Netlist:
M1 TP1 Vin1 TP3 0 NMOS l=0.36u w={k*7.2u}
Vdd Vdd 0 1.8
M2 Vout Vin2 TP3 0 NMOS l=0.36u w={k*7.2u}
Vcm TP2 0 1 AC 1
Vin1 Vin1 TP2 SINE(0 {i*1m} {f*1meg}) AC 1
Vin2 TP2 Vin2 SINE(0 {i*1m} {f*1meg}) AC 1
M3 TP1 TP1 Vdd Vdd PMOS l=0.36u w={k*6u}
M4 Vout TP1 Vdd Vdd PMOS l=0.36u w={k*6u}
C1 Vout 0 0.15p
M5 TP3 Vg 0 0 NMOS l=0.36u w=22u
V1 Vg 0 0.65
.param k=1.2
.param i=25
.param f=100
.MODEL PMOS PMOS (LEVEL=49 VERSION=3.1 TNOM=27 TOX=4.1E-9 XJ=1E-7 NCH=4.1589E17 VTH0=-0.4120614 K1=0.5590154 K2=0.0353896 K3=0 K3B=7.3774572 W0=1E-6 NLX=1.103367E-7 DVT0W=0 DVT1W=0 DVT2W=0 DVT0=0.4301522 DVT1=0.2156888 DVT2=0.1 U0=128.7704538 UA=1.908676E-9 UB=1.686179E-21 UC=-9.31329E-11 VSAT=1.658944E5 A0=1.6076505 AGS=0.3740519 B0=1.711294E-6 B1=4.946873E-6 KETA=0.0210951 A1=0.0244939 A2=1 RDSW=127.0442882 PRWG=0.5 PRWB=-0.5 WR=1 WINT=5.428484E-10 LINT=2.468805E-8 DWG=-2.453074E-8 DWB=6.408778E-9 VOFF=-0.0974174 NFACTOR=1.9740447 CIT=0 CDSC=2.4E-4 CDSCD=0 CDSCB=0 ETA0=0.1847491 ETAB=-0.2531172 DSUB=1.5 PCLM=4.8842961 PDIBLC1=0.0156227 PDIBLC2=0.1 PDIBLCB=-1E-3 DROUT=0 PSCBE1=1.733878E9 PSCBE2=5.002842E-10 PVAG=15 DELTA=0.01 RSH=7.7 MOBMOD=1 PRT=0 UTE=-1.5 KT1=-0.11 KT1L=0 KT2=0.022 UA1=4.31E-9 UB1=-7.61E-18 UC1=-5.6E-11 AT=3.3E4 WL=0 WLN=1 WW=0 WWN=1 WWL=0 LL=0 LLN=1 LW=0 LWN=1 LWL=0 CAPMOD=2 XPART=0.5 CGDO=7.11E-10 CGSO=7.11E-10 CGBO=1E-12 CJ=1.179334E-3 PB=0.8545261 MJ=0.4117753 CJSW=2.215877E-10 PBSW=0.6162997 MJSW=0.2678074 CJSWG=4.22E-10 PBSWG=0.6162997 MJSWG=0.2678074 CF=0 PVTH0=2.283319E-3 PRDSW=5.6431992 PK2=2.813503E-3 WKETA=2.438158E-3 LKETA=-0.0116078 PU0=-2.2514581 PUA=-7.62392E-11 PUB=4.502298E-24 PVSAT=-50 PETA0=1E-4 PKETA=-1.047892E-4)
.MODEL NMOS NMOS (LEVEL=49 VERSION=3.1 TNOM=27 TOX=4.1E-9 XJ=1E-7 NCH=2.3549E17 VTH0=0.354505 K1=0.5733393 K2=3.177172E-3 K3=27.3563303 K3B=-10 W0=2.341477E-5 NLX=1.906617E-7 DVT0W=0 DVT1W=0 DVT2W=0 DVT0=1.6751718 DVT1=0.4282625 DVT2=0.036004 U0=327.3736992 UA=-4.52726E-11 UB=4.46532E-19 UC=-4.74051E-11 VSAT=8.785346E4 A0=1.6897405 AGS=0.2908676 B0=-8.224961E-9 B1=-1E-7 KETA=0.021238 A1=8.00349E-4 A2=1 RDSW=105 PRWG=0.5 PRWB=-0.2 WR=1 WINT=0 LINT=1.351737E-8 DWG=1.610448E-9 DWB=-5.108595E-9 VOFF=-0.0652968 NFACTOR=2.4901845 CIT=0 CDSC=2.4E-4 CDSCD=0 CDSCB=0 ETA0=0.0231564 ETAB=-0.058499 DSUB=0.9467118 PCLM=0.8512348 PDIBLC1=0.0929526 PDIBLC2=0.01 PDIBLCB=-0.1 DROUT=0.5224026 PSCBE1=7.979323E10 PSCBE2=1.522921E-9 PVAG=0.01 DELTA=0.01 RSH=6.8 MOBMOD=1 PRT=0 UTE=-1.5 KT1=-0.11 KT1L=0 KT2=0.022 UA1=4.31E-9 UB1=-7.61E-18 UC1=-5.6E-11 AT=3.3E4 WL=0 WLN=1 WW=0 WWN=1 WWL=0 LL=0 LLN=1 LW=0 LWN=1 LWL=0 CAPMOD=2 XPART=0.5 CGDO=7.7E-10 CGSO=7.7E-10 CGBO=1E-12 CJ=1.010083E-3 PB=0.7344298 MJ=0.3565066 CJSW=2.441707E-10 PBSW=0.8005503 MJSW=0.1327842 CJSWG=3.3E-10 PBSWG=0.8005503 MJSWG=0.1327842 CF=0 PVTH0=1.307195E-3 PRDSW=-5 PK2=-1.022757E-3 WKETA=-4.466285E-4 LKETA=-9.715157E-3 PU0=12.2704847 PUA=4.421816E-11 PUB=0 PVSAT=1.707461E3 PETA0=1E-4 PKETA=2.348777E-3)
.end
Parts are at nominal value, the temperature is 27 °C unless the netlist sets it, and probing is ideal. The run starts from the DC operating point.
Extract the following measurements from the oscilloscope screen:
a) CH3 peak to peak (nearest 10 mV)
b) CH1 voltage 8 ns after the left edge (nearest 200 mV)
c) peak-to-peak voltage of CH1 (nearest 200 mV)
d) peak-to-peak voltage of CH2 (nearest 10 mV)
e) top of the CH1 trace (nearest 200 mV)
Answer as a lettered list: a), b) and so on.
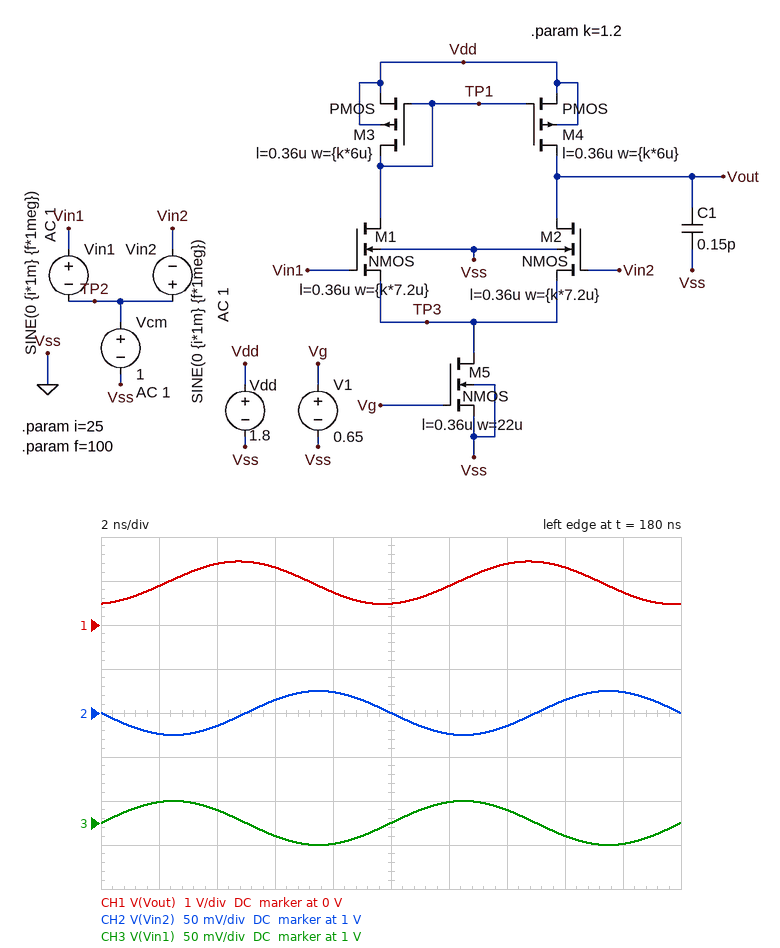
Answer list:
a) 50 mV
b) 800 mV
c) 1.0 V
d) 50 mV
e) 1.4 V
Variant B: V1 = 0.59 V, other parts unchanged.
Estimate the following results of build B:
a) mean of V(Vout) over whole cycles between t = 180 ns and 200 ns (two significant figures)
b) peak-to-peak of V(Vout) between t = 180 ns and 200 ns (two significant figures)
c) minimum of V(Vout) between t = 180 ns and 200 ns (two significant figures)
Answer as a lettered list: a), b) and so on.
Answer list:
a) 1.1 V
b) 600 mV
c) 780 mV
